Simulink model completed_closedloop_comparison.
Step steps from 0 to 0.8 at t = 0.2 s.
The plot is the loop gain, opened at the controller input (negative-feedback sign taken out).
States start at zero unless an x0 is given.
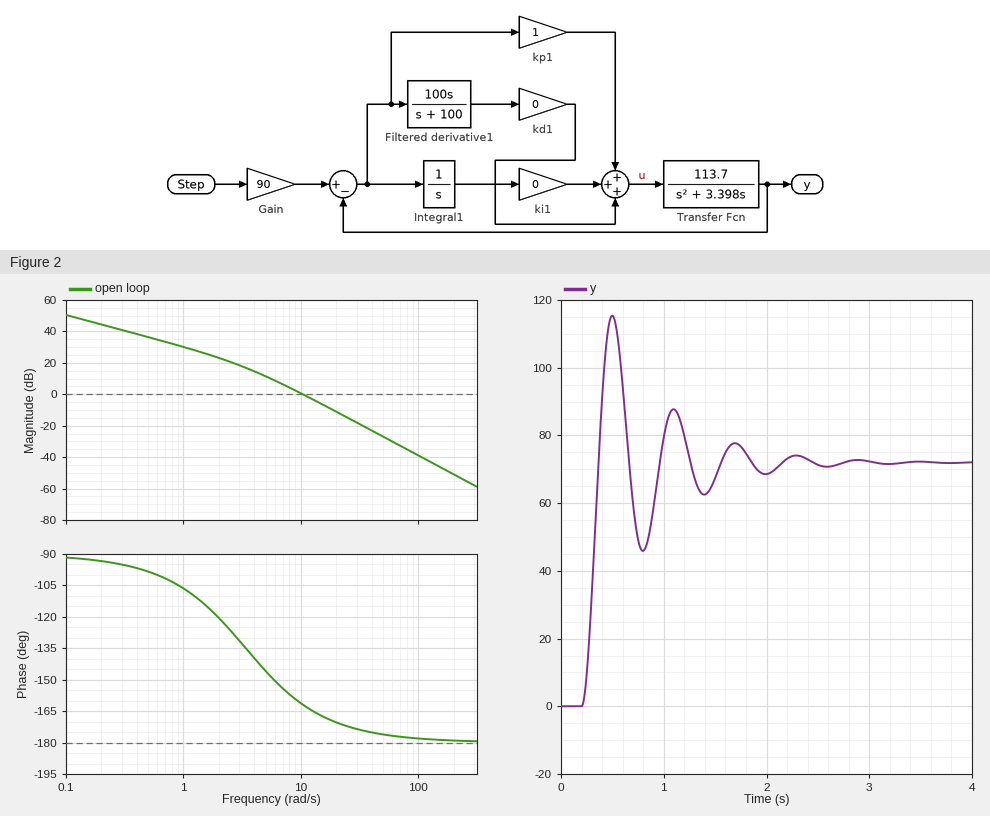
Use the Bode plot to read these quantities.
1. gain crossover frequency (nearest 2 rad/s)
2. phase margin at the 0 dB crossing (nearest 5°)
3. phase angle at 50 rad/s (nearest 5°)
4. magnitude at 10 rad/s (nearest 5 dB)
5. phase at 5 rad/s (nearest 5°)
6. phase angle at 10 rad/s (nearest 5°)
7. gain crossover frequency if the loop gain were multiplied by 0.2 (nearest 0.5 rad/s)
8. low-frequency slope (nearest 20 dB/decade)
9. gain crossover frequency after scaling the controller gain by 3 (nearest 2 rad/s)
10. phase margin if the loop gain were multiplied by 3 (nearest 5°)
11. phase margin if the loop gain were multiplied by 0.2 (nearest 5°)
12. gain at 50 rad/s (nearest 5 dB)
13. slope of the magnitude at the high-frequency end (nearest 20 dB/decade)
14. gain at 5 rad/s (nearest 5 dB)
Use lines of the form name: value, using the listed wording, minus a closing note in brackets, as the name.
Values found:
gain crossover frequency: 10 rad/s
phase margin at the 0 dB crossing: 20°
phase angle at 50 rad/s: -175°
magnitude at 10 rad/s: 0 dB
phase at 5 rad/s: -145°
phase angle at 10 rad/s: -160°
gain crossover frequency if the loop gain were multiplied by 0.2: 4.0 rad/s
low-frequency slope: -20 dB/decade
gain crossover frequency after scaling the controller gain by 3: 18 rad/s
phase margin if the loop gain were multiplied by 3: 10°
phase margin if the loop gain were multiplied by 0.2: 40°
gain at 50 rad/s: -25 dB
slope of the magnitude at the high-frequency end: -40 dB/decade
gain at 5 rad/s: 10 dB
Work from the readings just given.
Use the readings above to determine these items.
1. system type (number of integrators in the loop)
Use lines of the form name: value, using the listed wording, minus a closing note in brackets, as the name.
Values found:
system type: 1
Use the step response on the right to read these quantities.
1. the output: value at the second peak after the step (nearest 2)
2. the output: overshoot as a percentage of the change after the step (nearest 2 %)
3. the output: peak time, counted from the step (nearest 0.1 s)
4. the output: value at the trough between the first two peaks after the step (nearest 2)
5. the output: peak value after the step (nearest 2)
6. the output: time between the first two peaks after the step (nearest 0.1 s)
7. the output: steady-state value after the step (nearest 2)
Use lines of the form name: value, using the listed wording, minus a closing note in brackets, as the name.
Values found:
the output: value at the second peak after the step: 88
the output: overshoot as a percentage of the change after the step: 60 %
the output: peak time, counted from the step: 0.3 s
the output: value at the trough between the first two peaks after the step: 46
the output: peak value after the step: 116
the output: time between the first two peaks after the step: 0.6 s
the output: steady-state value after the step: 72
